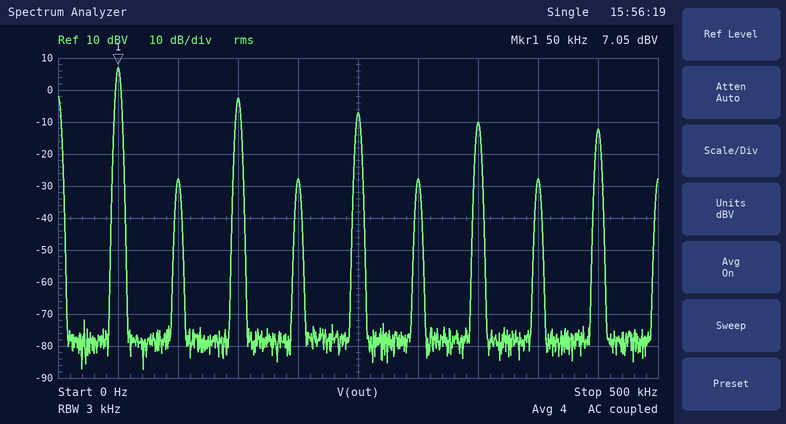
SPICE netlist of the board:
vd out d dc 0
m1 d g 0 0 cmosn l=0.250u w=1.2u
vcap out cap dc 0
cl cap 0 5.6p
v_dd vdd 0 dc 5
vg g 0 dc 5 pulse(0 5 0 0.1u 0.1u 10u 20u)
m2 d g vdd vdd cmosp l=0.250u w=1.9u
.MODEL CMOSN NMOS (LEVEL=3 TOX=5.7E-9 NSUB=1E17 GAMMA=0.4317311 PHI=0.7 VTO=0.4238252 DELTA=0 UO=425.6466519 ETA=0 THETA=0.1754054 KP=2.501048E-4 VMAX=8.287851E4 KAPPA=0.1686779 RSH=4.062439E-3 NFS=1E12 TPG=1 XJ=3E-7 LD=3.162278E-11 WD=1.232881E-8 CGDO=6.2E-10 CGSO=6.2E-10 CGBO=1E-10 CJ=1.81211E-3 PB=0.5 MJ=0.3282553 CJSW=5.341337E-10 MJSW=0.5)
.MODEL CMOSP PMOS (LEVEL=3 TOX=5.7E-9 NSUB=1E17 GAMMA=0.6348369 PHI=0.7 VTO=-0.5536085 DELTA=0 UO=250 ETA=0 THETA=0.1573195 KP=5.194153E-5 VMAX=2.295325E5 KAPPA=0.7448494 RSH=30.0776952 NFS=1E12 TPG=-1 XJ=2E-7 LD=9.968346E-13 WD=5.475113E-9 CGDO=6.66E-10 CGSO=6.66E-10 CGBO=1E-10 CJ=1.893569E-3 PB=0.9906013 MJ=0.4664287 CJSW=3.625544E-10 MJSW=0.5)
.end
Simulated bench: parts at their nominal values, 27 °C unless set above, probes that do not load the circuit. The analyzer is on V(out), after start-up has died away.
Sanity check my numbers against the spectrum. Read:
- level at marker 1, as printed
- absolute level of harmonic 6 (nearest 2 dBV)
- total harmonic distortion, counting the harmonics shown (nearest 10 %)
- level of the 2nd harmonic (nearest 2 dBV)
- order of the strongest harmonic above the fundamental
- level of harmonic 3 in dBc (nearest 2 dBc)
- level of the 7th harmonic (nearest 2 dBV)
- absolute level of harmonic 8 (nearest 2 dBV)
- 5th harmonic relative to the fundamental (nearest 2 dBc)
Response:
7.05 dBV
-28 dBV
40 %
-28 dBV
3
-10 dBc
-10 dBV
-28 dBV
-14 dBc
